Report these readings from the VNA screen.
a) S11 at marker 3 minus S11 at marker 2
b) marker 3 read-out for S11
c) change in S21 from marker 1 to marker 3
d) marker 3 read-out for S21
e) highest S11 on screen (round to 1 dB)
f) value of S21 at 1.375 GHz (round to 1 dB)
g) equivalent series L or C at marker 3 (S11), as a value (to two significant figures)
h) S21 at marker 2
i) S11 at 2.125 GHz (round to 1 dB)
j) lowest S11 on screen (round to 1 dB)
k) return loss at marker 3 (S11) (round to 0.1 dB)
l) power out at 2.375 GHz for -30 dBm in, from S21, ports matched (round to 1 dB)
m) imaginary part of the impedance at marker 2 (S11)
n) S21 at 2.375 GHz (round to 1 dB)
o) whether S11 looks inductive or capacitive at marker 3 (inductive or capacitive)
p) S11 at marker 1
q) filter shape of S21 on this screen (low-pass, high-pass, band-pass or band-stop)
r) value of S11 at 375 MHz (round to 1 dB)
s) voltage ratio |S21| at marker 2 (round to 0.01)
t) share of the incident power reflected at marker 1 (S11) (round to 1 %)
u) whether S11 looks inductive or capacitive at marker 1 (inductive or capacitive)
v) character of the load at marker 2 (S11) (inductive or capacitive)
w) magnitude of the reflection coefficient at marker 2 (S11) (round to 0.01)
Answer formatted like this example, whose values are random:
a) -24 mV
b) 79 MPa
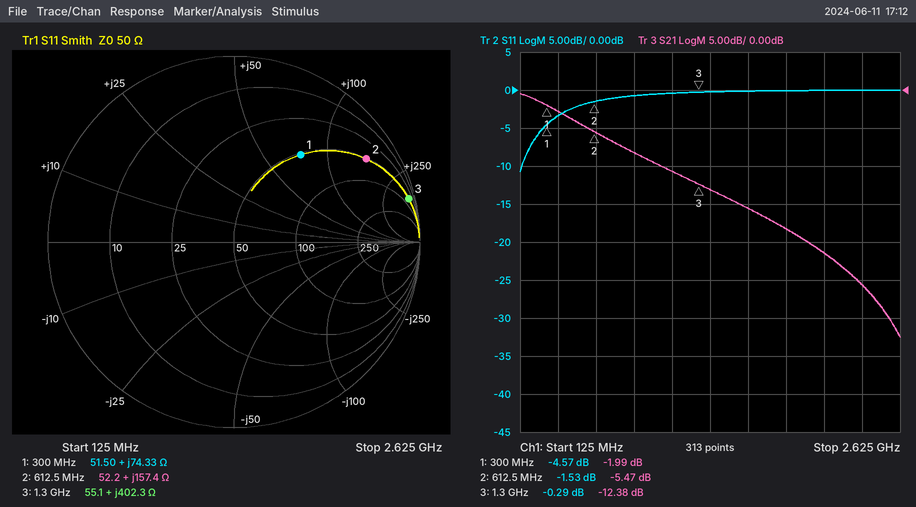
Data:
a) 1.24 dB
b) -0.29 dB
c) -10.39 dB
d) -12.38 dB
e) 0 dB
f) -13 dB
g) 49 nH
h) -5.47 dB
i) 0 dB
j) -11 dB
k) 0.3 dB
l) -56 dBm
m) +157.4 Ω
n) -26 dB
o) inductive
p) -4.57 dB
q) low-pass
r) -3 dB
s) 0.53
t) 35 %
u) inductive
v) inductive
w) 0.84
